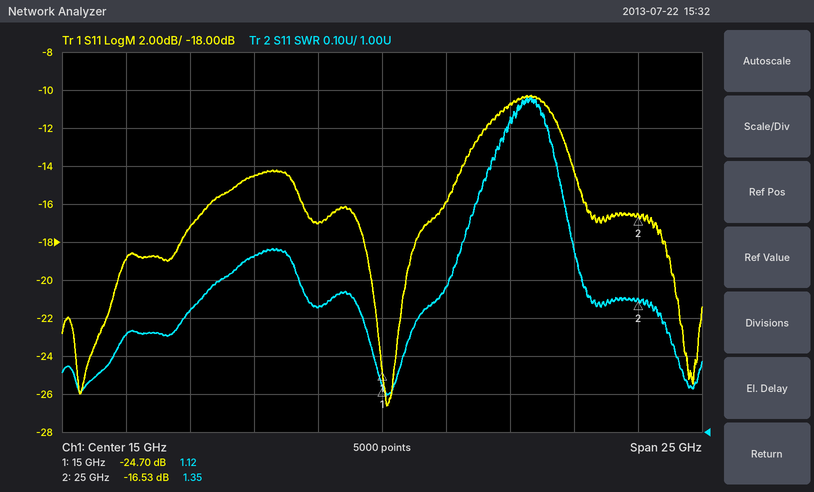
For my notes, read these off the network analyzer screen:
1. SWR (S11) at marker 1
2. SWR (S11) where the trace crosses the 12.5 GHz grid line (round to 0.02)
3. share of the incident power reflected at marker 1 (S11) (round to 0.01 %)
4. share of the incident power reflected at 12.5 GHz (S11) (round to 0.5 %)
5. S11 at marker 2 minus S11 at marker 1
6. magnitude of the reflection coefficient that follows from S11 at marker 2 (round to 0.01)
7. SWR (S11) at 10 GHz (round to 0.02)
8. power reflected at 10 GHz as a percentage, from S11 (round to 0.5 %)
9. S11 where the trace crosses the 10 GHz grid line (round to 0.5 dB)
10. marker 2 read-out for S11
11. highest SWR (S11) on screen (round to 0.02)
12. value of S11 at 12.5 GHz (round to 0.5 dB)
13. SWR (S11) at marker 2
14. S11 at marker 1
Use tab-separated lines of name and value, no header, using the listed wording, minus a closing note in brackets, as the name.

SWR (S11) at marker 1	1.12
SWR (S11) where the trace crosses the 12.5 GHz grid line	1.32
share of the incident power reflected at marker 1 (S11)	0.34 %
share of the incident power reflected at 12.5 GHz (S11)	2.0 %
S11 at marker 2 minus S11 at marker 1	8.17 dB
magnitude of the reflection coefficient that follows from S11 at marker 2	0.15
SWR (S11) at 10 GHz	1.46
power reflected at 10 GHz as a percentage, from S11	3.5 %
S11 where the trace crosses the 10 GHz grid line	-14.5 dB
marker 2 read-out for S11	-16.53 dB
highest SWR (S11) on screen	1.88
value of S11 at 12.5 GHz	-17.0 dB
SWR (S11) at marker 2	1.35
S11 at marker 1	-24.70 dB
